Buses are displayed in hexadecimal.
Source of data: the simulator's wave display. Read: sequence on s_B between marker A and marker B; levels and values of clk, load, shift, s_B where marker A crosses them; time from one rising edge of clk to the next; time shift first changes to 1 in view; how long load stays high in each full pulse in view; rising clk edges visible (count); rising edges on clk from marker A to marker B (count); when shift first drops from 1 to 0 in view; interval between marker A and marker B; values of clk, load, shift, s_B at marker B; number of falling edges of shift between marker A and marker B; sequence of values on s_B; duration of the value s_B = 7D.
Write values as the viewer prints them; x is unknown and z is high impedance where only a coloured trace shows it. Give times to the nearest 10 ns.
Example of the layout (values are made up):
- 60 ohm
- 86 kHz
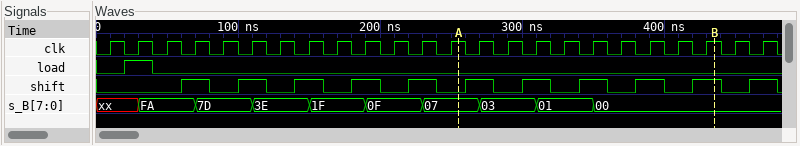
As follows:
- 07, 03, 01, 00
- clk=1, load=0, shift=0, s_B=07
- 20 ns
- 60 ns
- 20 ns
- 24
- 9
- 80 ns
- 180 ns
- clk=1, load=0, shift=1, s_B=00
- 4
- xx, FA, 7D, 3E, 1F, 0F, 07, 03, 01, 00
- 40 ns
